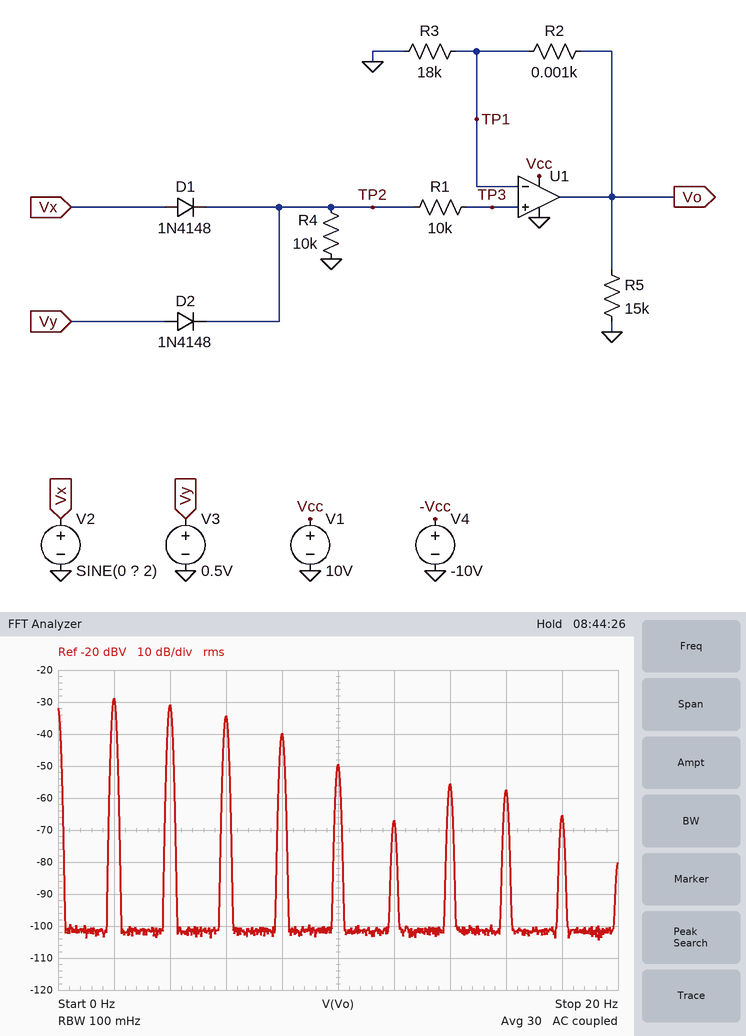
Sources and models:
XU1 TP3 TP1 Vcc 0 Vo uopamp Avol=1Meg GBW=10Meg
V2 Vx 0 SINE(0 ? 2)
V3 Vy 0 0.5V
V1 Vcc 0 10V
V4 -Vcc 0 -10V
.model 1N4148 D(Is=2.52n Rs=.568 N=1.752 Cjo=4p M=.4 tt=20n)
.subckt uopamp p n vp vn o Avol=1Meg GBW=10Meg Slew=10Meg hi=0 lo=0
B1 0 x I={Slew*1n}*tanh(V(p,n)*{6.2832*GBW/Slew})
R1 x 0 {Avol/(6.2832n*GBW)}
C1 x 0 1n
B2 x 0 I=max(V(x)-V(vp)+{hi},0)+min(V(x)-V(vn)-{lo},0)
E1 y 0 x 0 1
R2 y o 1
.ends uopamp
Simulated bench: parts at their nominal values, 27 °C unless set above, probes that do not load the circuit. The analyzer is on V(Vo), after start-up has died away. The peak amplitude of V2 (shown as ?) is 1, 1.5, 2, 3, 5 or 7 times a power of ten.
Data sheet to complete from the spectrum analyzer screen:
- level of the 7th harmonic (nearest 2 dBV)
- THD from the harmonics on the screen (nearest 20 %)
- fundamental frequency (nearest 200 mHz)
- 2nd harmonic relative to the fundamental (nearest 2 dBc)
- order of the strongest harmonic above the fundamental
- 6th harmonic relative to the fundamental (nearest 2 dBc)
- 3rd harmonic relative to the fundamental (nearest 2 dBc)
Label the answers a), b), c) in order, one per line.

a) -56 dBV
b) 100 %
c) 2.0 Hz
d) -2 dBc
e) 2
f) -38 dBc
g) -6 dBc
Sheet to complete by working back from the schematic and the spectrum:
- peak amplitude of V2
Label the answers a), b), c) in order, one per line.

a) 700 mV
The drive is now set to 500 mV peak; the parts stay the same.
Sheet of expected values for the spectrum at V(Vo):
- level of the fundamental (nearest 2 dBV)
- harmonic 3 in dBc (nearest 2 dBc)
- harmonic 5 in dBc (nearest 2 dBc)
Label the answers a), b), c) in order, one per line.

a) -48 dBV
b) -4 dBc
c) -12 dBc
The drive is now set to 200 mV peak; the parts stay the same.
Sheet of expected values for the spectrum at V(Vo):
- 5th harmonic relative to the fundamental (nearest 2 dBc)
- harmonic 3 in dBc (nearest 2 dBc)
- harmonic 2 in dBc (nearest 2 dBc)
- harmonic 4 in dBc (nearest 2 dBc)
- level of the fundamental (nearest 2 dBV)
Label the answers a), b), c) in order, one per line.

a) -24 dBc
b) -8 dBc
c) -4 dBc
d) -16 dBc
e) -100 dBV
